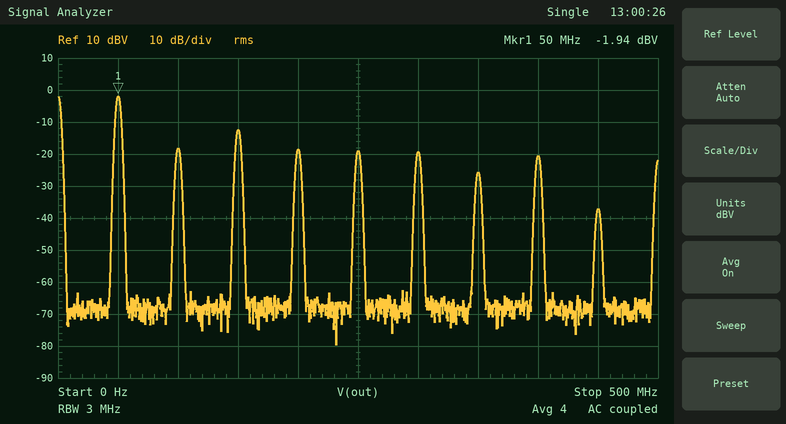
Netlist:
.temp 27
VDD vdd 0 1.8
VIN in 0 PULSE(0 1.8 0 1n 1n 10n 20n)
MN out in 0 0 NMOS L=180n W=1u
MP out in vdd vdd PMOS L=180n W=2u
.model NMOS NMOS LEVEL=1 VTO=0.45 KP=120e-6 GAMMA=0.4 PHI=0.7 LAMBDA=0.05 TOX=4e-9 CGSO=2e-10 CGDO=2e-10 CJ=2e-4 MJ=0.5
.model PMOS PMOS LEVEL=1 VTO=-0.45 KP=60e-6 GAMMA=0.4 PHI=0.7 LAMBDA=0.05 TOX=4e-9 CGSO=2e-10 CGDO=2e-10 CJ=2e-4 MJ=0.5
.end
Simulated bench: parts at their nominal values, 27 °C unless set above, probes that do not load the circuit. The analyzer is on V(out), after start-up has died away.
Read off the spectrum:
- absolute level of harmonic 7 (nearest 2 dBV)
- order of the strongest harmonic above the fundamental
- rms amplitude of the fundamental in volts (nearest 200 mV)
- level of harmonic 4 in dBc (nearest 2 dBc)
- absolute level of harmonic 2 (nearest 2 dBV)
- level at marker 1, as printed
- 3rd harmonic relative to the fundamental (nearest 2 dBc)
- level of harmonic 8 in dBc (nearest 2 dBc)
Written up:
-26 dBV
3
800 mV
-16 dBc
-18 dBV
-1.94 dBV
-10 dBc
-18 dBc
